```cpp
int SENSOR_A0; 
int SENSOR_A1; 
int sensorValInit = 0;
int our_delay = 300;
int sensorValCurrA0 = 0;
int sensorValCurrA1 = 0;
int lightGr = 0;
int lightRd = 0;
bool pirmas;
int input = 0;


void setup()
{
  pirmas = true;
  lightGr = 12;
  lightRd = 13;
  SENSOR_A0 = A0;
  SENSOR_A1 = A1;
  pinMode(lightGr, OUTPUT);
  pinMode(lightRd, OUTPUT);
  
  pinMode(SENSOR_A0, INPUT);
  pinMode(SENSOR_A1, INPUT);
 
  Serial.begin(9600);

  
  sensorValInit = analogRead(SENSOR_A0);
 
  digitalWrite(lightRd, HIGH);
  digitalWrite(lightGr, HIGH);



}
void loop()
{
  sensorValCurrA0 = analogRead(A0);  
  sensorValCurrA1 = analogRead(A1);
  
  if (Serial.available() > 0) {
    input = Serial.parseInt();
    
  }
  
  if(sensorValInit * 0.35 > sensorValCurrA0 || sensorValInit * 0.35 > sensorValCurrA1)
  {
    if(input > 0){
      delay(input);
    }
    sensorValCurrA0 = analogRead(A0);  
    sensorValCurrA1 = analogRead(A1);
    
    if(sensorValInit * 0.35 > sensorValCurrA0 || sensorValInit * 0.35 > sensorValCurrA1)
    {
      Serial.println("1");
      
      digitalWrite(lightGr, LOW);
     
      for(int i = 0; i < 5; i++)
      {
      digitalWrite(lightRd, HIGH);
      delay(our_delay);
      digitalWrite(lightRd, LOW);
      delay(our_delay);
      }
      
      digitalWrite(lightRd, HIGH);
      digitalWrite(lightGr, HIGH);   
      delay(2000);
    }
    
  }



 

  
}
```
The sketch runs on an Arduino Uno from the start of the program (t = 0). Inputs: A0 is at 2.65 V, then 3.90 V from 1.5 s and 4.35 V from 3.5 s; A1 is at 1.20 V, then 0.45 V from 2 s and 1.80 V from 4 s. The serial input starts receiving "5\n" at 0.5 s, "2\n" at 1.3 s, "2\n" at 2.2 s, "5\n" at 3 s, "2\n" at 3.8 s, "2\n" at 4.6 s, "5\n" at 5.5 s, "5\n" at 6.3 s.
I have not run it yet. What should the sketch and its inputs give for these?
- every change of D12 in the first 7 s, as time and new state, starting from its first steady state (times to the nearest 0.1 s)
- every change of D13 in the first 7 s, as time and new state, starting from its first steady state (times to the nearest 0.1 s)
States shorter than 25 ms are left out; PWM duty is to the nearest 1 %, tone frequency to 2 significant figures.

0 s high; 3 s low; 6 s high
0 s high; 3.3 s low; 3.6 s high; 3.9 s low; 4.2 s high; 4.5 s low; 4.8 s high; 5.1 s low; 5.4 s high; 5.7 s low; 6 s high
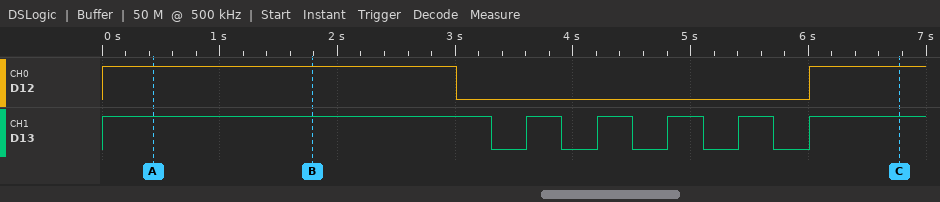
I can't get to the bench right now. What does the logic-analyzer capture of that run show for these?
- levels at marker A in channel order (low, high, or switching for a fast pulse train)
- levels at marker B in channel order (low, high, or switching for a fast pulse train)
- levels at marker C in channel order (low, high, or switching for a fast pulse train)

D12 high, D13 high
D12 high, D13 high
D12 high, D13 high
